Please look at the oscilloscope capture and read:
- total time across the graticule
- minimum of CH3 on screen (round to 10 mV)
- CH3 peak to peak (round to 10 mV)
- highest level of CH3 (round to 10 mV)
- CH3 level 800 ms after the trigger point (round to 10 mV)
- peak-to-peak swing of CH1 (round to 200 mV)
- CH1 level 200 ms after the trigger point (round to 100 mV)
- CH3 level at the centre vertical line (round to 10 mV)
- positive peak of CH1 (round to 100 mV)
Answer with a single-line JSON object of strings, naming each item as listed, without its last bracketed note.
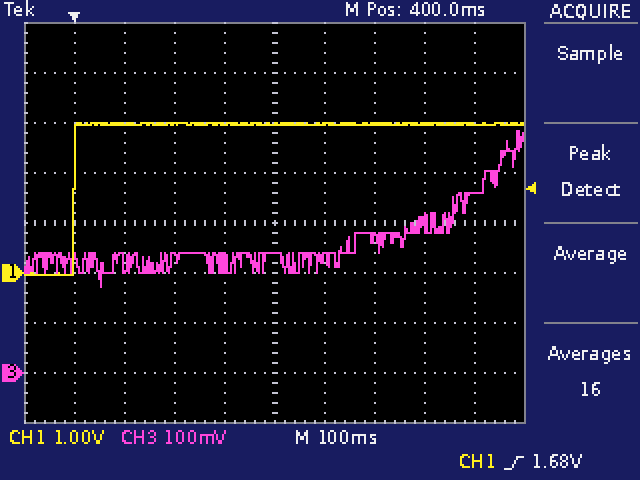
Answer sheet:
{"total time across the graticule": "1 s", "minimum of CH3 on screen": "170 mV", "CH3 peak to peak": "310 mV", "highest level of CH3": "480 mV", "CH3 level 800 ms after the trigger point": "360 mV", "peak-to-peak swing of CH1": "3.0 V", "CH1 level 200 ms after the trigger point": "3.0 V", "CH3 level at the centre vertical line": "240 mV", "positive peak of CH1": "3.0 V"}
